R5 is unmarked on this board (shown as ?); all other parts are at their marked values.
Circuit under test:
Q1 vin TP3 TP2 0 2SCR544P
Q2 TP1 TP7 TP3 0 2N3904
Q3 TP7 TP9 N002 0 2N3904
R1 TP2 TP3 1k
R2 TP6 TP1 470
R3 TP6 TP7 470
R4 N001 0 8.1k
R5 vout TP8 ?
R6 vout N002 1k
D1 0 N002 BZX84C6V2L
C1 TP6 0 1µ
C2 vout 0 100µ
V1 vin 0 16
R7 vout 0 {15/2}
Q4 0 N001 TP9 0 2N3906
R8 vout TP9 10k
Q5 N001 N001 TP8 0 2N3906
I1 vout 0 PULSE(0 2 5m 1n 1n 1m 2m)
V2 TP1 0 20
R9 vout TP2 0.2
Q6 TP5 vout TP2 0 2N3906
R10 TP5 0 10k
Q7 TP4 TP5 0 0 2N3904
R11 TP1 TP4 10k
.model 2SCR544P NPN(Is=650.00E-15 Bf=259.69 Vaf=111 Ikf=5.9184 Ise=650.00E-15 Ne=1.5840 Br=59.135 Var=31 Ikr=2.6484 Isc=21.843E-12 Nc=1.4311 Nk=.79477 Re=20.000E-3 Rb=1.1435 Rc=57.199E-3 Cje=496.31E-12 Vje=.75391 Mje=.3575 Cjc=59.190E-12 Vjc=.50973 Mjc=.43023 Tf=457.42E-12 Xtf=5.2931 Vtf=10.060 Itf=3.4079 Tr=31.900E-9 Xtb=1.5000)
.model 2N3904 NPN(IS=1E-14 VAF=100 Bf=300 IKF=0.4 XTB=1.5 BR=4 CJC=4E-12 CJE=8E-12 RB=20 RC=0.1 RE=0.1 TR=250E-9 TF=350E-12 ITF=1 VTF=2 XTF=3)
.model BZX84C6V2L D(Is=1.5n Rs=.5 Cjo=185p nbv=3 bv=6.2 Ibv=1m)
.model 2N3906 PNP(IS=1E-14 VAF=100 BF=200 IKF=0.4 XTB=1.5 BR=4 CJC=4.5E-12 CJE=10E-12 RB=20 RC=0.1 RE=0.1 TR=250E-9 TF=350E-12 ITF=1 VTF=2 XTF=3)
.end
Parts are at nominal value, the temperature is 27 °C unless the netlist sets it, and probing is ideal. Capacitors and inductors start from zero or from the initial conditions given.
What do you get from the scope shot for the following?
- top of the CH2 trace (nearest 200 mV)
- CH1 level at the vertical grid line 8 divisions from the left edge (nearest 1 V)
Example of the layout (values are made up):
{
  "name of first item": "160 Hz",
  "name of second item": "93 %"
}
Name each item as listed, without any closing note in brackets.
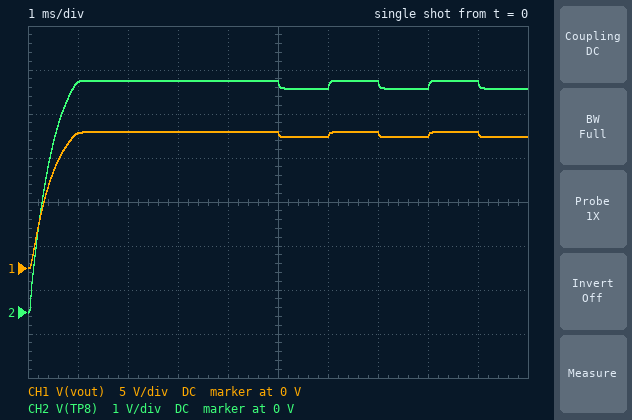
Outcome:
{
  "top of the CH2 trace": "5.2 V",
  "CH1 level at the vertical grid line 8 divisions from the left edge": "15 V"
}
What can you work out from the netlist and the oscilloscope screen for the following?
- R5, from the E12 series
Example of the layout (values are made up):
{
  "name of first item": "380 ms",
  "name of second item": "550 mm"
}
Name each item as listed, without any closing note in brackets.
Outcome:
{
  "R5, from the E12 series": "18 kΩ"
}
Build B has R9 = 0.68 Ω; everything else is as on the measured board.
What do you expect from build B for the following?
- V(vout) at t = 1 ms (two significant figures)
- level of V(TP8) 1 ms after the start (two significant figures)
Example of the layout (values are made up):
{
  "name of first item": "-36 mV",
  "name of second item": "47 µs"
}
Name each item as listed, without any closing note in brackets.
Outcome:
{
  "V(vout) at t = 1 ms": "14 V",
  "level of V(TP8) 1 ms after the start": "4.9 V"
}
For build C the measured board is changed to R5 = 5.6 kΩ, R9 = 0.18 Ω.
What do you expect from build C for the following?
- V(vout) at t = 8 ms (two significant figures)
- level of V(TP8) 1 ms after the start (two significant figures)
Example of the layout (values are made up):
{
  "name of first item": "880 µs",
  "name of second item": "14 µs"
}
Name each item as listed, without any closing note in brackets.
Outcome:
{
  "V(vout) at t = 8 ms": "12 V",
  "level of V(TP8) 1 ms after the start": "7.1 V"
}
